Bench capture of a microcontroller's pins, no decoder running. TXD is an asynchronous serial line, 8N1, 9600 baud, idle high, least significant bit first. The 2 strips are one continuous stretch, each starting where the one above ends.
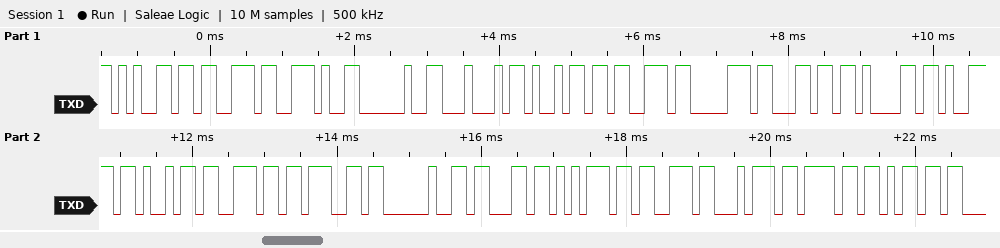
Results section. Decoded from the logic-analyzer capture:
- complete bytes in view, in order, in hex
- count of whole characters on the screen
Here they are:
65 73 2E 20 44 69 73 70 6C 61 79 69 6E 67 20 63 75 73 74 6F 6D
21
